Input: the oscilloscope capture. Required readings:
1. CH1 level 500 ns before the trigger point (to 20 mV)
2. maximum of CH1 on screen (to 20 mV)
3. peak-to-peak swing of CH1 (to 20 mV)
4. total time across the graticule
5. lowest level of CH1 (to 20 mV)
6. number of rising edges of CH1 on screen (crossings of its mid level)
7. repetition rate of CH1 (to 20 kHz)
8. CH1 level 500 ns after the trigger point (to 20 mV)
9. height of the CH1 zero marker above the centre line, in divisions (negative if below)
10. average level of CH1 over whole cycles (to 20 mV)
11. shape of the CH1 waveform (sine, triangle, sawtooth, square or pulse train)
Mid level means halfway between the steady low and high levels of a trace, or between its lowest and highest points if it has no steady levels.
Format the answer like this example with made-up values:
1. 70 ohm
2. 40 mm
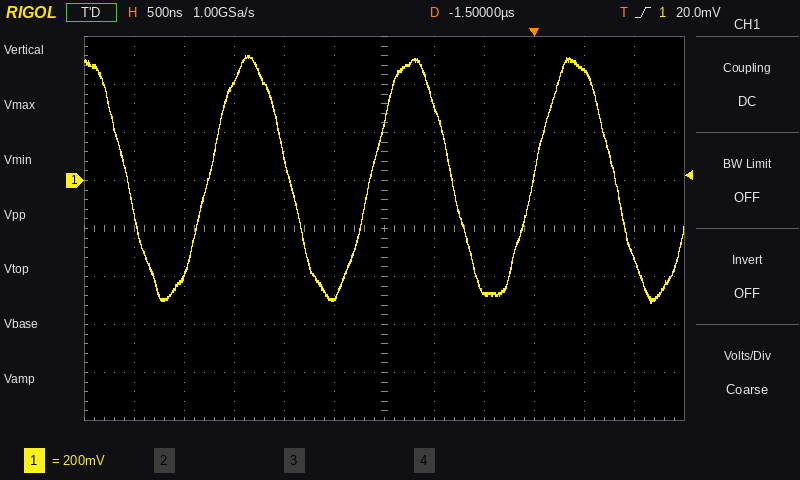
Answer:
1. -460 mV
2. 520 mV
3. 1.04 V
4. 6 µs
5. -520 mV
6. 3
7. 620 kHz
8. 460 mV
9. +1.0 div
10. 0 mV
11. sine
